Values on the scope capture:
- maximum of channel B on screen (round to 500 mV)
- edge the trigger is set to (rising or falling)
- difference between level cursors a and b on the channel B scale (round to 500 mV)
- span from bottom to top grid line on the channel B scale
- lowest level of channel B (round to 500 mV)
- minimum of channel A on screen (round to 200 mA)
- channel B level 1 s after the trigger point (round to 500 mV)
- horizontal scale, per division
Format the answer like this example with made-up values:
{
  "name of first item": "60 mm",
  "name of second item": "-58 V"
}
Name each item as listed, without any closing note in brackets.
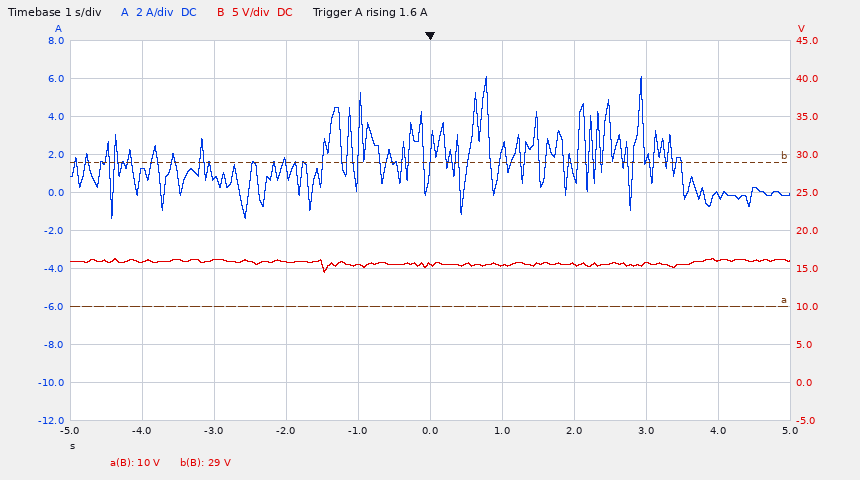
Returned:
{
  "maximum of channel B on screen": "16.5 V",
  "edge the trigger is set to": "rising",
  "difference between level cursors a and b on the channel B scale": "19.0 V",
  "span from bottom to top grid line on the channel B scale": "50 V",
  "lowest level of channel B": "14.5 V",
  "minimum of channel A on screen": "-1.4 A",
  "channel B level 1 s after the trigger point": "15.5 V",
  "horizontal scale, per division": "1 s"
}
